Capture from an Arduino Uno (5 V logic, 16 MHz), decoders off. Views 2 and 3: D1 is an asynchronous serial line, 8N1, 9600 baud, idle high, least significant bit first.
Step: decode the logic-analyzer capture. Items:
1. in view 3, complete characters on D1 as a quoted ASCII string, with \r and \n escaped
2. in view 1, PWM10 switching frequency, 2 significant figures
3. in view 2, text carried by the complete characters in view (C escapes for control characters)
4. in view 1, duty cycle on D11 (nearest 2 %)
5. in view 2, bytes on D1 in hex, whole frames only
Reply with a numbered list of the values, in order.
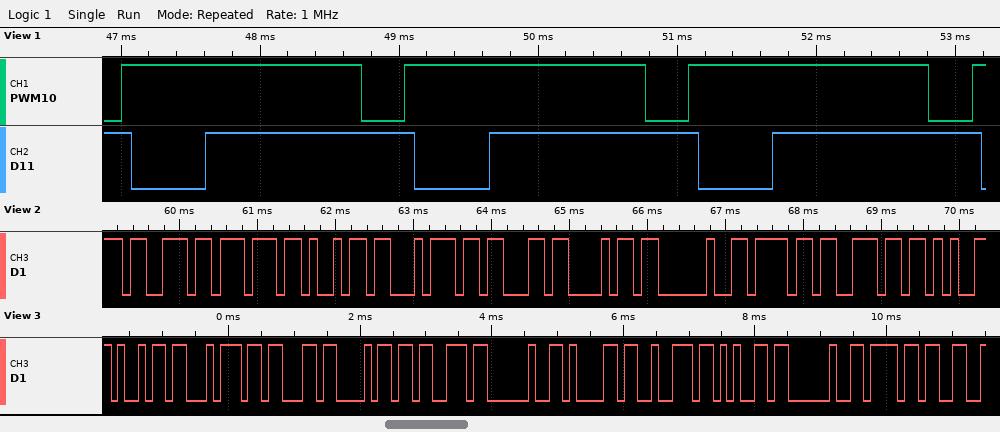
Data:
1. "itchs are o"
2. 490 Hz
3. "switch on"
4. 74 %
5. 73 77 69 74 63 68 20 6F 6E
